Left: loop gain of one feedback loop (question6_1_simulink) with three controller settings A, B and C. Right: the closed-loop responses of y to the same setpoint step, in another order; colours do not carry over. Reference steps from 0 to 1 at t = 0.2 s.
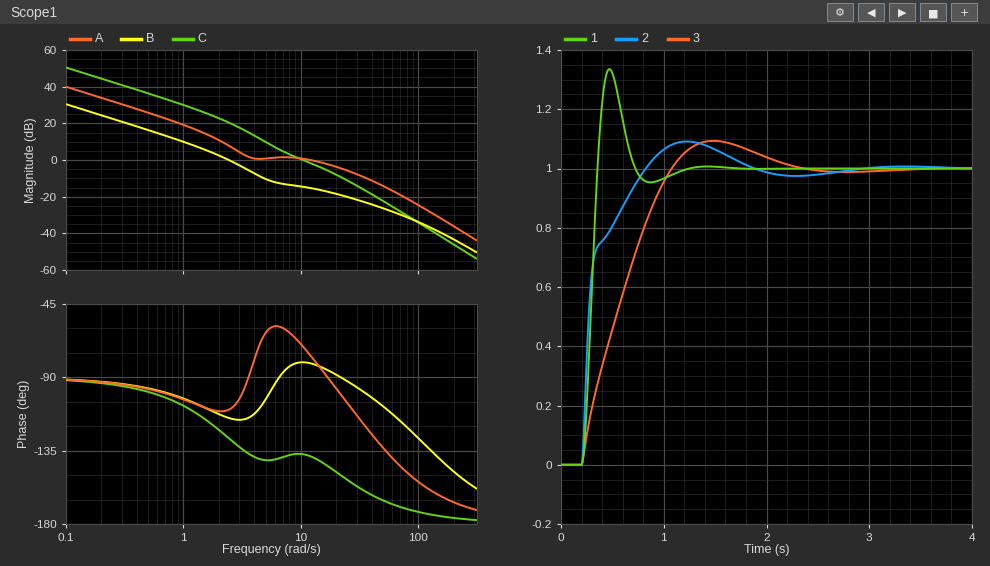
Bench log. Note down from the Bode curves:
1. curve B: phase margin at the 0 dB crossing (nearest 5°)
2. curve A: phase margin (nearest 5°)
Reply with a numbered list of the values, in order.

1. 65°
2. 105°
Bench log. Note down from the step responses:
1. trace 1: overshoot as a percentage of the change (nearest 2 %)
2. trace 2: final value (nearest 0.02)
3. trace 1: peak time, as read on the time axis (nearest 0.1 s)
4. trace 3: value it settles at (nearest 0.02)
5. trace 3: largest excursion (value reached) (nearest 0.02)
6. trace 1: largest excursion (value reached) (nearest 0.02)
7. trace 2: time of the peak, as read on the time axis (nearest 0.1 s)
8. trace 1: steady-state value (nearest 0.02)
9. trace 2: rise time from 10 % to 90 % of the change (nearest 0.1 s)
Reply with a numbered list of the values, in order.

1. 34 %
2. 1.00
3. 0.5 s
4. 1.00
5. 1.10
6. 1.34
7. 1.2 s
8. 1.00
9. 0.4 s
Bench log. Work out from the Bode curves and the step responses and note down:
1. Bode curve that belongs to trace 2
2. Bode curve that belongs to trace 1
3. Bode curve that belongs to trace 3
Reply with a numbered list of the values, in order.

1. A
2. C
3. B
